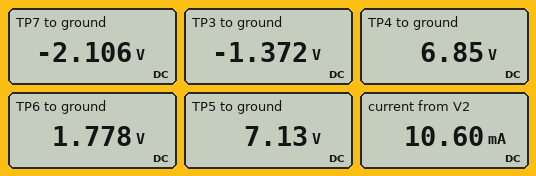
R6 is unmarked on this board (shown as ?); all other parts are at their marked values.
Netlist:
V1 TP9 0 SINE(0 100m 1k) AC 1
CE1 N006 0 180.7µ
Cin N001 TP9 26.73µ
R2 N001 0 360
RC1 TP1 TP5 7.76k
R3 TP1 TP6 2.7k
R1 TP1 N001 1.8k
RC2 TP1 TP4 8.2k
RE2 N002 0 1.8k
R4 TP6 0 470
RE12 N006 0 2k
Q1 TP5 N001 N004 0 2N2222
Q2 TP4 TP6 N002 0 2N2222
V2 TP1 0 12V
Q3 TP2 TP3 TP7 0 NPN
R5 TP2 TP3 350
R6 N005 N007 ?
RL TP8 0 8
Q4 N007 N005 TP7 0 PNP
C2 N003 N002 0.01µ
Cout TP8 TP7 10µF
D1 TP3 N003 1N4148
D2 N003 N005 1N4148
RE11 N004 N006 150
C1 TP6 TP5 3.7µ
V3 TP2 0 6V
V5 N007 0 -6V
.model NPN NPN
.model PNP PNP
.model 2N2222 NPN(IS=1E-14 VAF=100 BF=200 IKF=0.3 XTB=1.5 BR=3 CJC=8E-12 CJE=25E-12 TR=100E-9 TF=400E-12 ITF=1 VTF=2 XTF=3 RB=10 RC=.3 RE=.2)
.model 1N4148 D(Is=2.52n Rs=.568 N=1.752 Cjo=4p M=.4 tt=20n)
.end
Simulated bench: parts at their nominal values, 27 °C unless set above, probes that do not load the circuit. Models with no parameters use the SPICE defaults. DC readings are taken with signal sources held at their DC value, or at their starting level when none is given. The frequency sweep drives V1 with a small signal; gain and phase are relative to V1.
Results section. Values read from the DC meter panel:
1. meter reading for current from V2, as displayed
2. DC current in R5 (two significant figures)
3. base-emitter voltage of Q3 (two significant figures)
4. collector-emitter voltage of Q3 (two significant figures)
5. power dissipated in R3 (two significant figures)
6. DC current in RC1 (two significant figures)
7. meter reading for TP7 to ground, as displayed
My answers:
10.60 mA
21 mA
730 mV
8.1 V
39 mW
630 µA
-2.106 V
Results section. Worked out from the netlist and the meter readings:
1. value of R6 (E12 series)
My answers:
150 Ω
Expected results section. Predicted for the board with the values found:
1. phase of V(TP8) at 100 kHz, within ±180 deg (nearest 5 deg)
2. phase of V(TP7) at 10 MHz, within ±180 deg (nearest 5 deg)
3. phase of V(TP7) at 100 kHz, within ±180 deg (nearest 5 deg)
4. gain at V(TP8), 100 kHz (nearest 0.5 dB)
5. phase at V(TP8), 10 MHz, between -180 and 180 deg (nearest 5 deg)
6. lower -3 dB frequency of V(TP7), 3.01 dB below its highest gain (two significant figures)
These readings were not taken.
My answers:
-135 deg
150 deg
-135 deg
-19.0 dB
150 deg
97 kHz
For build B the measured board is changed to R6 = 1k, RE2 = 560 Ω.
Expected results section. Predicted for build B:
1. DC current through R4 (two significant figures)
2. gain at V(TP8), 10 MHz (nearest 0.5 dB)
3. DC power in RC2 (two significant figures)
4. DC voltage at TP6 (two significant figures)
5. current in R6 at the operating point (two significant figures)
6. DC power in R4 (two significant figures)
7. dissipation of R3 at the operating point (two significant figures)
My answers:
3.5 mA
-39.5 dB
15 mW
1.6 V
7.9 mA
5.7 mW
40 mW
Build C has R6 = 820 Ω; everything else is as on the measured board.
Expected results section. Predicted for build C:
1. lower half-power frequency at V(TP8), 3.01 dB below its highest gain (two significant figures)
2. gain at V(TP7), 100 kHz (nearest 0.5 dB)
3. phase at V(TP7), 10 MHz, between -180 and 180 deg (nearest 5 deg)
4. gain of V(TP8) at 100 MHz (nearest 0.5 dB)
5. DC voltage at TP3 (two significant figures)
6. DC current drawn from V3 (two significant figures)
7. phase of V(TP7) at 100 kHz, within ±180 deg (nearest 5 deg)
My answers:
53 kHz
-29.5 dB
155 deg
-36.5 dB
2.8 V
9.1 mA
-155 deg
